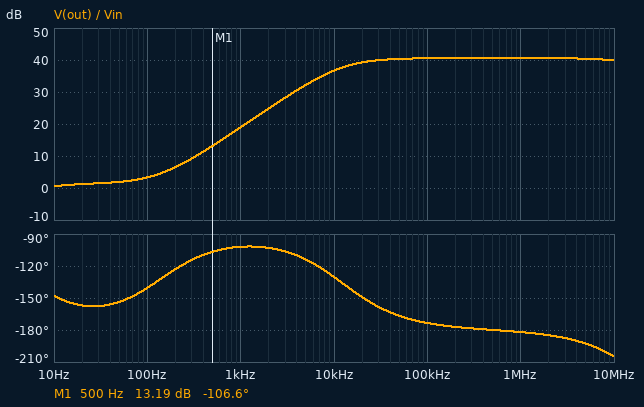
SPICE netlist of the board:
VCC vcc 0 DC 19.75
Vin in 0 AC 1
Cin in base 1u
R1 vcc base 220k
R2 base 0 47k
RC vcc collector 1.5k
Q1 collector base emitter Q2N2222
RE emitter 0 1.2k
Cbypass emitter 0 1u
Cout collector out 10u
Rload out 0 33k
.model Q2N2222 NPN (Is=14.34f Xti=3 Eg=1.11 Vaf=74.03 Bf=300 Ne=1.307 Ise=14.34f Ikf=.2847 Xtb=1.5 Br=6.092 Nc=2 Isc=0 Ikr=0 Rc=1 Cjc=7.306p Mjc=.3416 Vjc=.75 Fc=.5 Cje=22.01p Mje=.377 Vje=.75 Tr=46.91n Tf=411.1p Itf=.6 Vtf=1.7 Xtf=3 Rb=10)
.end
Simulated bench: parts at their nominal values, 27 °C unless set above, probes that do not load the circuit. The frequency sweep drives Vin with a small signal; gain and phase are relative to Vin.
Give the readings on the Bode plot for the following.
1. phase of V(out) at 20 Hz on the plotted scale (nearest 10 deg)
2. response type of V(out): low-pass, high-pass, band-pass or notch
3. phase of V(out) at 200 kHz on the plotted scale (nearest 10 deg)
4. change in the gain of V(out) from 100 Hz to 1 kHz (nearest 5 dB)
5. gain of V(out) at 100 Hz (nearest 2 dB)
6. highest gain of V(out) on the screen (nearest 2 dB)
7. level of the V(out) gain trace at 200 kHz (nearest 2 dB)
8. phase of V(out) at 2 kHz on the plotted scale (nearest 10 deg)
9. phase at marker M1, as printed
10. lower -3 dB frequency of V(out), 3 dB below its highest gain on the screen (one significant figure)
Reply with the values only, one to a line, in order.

-160 deg
high-pass
-180 deg
15 dB
4 dB
40 dB
40 dB
-100 deg
-106.6 deg
10 kHz
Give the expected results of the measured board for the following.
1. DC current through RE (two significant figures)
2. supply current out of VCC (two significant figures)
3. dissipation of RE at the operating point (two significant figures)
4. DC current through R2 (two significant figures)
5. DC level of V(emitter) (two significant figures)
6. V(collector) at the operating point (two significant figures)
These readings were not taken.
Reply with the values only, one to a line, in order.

2.0 mA
2.1 mA
4.9 mW
66 µA
2.4 V
17 V
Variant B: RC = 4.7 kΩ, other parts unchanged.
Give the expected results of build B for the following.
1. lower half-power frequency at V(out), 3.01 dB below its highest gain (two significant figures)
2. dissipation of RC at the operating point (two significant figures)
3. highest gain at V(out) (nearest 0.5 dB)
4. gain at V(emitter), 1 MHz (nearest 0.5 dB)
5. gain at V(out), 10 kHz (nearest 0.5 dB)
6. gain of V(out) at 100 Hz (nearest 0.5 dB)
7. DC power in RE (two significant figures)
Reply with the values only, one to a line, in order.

11 kHz
19 mW
49.0 dB
-39.0 dB
45.5 dB
12.5 dB
4.8 mW
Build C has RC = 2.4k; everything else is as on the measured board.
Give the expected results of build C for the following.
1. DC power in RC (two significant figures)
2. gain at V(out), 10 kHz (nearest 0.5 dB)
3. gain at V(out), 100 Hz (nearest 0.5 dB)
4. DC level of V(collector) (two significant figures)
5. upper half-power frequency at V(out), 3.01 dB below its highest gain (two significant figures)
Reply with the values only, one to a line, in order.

9.7 mW
40.5 dB
7.0 dB
15 V
15 MHz
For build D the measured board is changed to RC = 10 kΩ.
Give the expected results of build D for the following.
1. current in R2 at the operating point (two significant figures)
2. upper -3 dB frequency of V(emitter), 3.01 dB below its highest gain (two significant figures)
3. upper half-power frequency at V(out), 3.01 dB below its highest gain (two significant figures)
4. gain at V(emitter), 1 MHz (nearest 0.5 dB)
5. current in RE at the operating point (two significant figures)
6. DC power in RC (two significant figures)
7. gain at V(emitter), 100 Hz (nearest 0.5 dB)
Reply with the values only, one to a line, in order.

59 µA
3.6 kHz
2.4 MHz
-50.0 dB
1.8 mA
31 mW
-6.5 dB
